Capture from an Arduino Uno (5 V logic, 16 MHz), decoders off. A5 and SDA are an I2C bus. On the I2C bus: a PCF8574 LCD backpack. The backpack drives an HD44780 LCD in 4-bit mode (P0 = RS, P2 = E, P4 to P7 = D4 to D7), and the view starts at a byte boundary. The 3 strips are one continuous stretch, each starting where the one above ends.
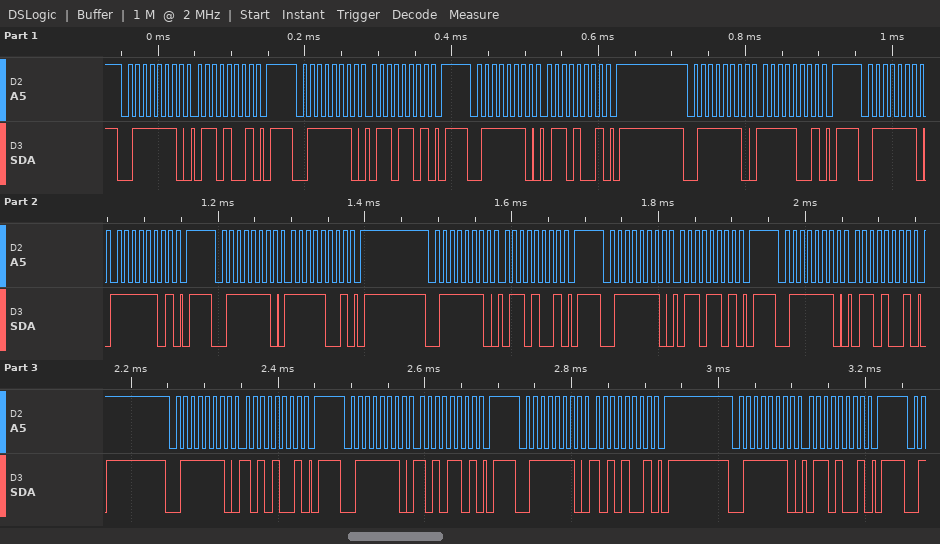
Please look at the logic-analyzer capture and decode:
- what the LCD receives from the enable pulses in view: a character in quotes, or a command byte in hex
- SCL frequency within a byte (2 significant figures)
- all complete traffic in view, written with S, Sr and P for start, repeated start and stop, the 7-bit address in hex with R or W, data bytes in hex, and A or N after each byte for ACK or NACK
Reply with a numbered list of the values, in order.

1. 'o' 'j'
2. 100 kHz
3. S 3FW A 69 A P S 3FW A 6D A P S 3FW A 69 A P S 3FW A F9 A P S 3FW A FD A P S 3FW A F9 A P S 3FW A 69 A P S 3FW A 6D A P S 3FW A 69 A P S 3FW A A9 A P S 3FW A AD A P S 3FW A A9 A P S 3FW A 69 A P
